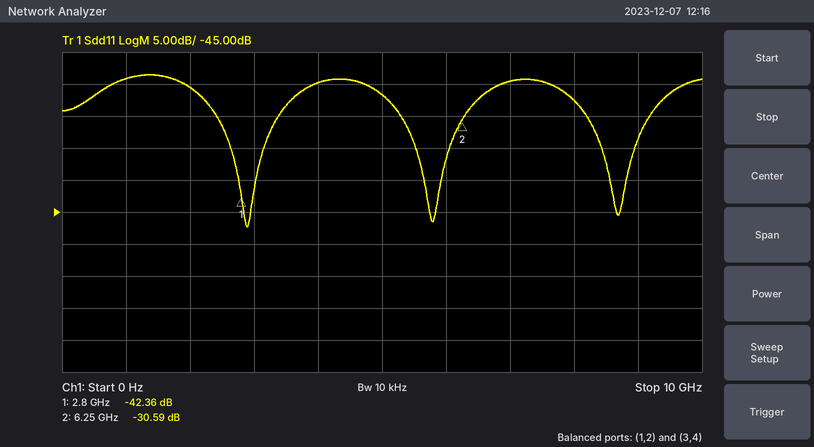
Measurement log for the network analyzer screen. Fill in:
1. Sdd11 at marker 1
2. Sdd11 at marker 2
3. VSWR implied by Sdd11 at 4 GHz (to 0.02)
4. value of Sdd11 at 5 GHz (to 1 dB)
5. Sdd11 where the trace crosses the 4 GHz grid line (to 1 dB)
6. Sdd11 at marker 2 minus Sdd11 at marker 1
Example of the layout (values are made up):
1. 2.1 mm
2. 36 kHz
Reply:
1. -42.36 dB
2. -30.59 dB
3. 1.12
4. -27 dB
5. -25 dB
6. 11.77 dB
